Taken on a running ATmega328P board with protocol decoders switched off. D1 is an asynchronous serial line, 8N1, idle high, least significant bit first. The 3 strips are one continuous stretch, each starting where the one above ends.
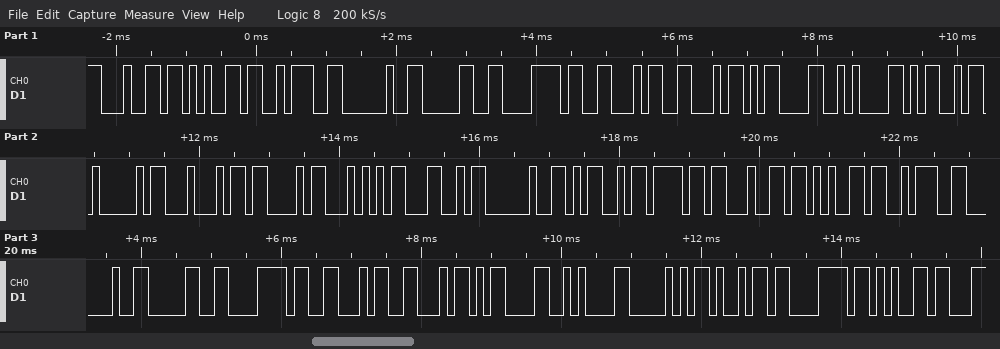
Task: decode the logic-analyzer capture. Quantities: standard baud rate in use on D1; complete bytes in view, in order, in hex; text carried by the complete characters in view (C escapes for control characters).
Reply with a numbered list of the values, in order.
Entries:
1. 9600 baud
2. 64 65 3A 20 30 78 46 46 0D 0A 4D 41 44 43 54 4C 20 4D 6F 64 65 3A 20 30 78 46 46 0D 0A 50 69 78 65
3. "de: 0xFF\r\nMADCTL Mode: 0xFF\r\nPixe"
